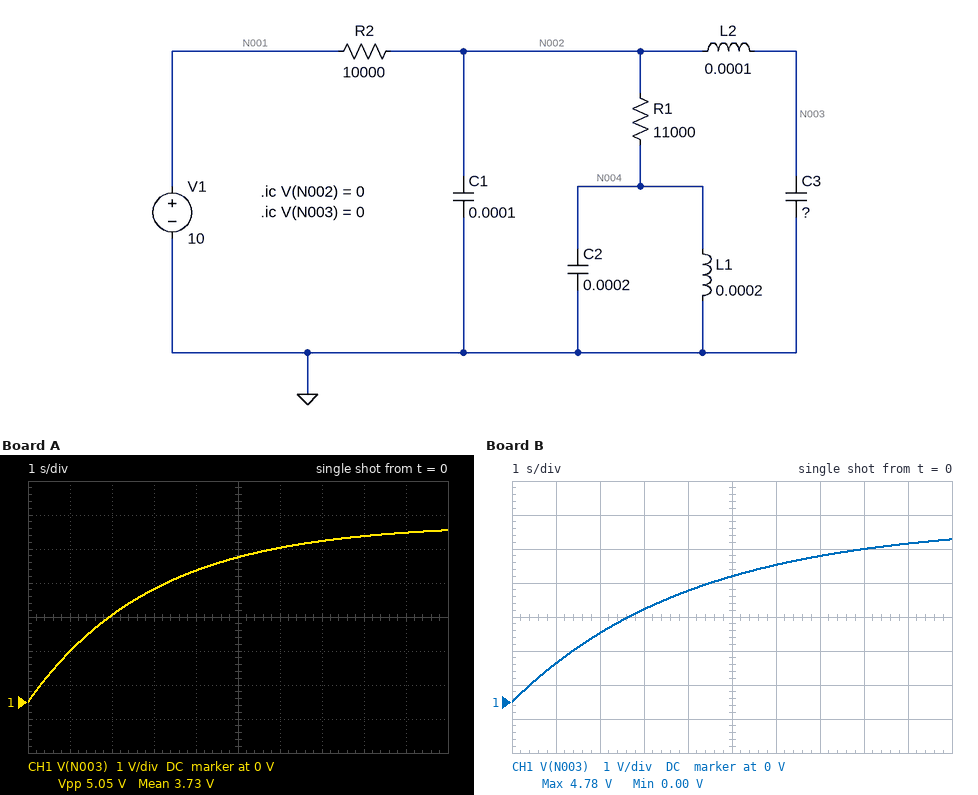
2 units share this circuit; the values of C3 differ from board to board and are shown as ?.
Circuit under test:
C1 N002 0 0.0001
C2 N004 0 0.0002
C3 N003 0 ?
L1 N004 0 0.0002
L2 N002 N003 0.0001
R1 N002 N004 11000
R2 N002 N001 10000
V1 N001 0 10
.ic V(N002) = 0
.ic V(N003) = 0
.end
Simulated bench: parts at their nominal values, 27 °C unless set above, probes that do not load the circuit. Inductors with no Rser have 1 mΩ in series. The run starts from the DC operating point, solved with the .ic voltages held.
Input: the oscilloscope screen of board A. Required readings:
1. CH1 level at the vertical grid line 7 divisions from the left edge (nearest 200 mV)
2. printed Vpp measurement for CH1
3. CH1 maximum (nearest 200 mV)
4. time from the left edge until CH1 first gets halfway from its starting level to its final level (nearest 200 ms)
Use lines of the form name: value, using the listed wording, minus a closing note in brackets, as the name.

CH1 level at the vertical grid line 7 divisions from the left edge: 4.8 V
printed Vpp measurement for CH1: 5.05 V
CH1 maximum: 5.0 V
time from the left edge until CH1 first gets halfway from its starting level to its final level: 2.0 s
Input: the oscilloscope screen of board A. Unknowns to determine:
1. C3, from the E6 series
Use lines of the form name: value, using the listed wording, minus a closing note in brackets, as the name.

C3, from the E6 series: 470 µF
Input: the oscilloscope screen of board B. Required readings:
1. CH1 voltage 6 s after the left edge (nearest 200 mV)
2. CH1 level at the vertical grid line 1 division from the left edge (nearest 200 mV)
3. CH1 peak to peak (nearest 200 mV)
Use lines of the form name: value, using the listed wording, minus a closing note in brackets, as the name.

CH1 voltage 6 s after the left edge: 4.0 V
CH1 level at the vertical grid line 1 division from the left edge: 1.2 V
CH1 peak to peak: 4.8 V
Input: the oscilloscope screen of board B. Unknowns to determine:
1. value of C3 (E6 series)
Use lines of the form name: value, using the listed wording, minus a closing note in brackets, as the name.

value of C3: 680 µF
